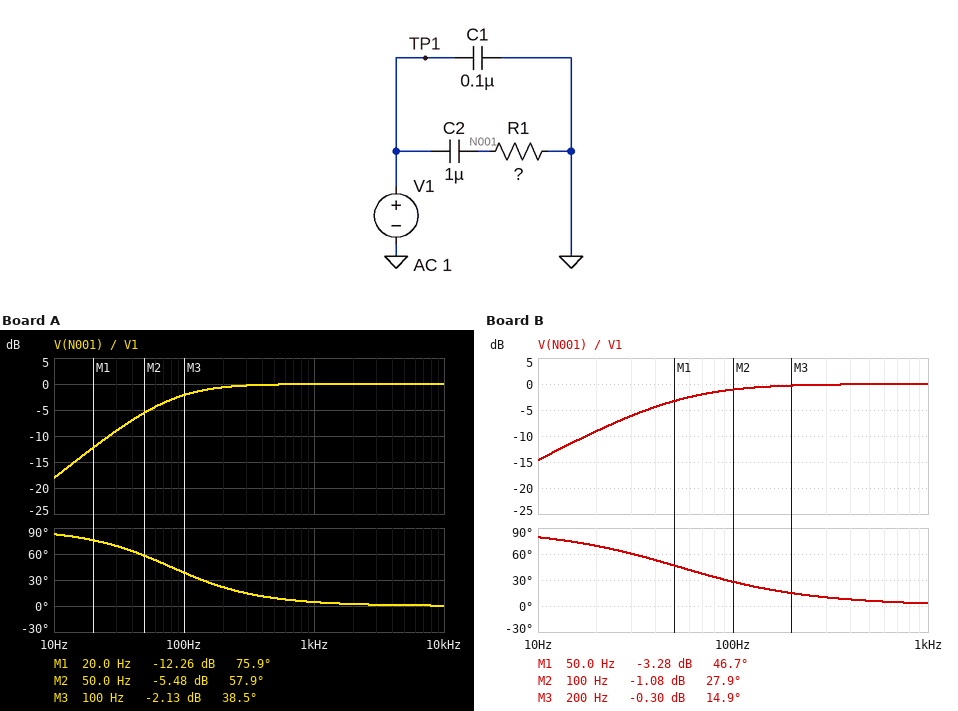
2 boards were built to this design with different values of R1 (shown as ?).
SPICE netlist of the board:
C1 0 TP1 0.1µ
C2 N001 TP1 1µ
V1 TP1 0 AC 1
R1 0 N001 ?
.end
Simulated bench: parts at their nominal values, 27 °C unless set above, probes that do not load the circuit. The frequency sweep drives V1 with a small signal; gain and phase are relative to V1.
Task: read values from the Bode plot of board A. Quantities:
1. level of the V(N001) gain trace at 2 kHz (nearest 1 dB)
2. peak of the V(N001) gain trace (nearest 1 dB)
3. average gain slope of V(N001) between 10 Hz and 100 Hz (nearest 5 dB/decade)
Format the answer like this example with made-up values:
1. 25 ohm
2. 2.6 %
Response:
1. 0 dB
2. 0 dB
3. 15 dB/decade
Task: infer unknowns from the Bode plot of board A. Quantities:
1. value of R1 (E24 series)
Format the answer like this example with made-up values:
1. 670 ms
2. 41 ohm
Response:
1. 2 kΩ
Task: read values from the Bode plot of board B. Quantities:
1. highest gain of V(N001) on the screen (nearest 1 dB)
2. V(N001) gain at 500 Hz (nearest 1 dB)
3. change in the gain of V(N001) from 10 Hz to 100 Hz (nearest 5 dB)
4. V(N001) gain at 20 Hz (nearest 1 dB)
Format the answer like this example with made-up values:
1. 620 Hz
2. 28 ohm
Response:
1. 0 dB
2. 0 dB
3. 15 dB
4. -9 dB
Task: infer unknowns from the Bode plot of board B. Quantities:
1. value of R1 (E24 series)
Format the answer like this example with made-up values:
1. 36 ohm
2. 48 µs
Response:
1. 3 kΩ
